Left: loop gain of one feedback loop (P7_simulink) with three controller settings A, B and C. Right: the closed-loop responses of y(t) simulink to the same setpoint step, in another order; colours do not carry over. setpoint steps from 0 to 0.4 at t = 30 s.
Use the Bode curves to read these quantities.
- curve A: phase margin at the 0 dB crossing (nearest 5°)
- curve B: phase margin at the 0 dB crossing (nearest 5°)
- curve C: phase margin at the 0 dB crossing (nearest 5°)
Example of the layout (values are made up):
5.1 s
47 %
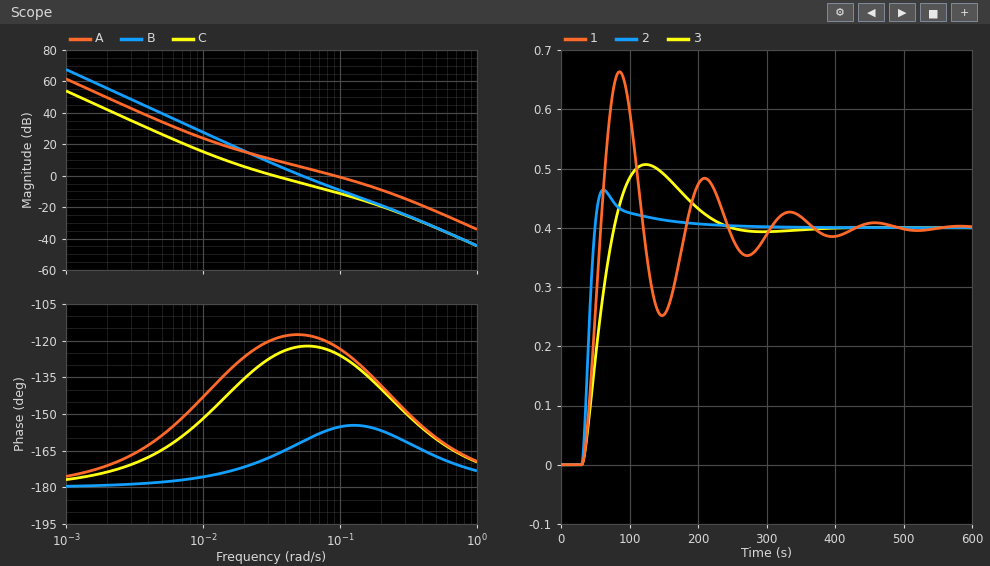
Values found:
60°
20°
55°
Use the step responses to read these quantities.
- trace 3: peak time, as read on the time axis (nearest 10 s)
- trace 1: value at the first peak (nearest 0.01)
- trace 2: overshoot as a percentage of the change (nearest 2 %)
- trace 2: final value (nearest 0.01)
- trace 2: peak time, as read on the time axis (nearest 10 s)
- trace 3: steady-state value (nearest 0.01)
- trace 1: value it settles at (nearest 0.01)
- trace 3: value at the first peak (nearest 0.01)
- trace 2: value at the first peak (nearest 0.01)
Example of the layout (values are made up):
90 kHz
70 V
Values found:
120 s
0.66
16 %
0.40
60 s
0.40
0.40
0.51
0.46
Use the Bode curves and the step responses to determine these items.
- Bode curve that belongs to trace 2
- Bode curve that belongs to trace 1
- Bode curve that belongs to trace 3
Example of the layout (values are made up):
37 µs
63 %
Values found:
A
B
C
